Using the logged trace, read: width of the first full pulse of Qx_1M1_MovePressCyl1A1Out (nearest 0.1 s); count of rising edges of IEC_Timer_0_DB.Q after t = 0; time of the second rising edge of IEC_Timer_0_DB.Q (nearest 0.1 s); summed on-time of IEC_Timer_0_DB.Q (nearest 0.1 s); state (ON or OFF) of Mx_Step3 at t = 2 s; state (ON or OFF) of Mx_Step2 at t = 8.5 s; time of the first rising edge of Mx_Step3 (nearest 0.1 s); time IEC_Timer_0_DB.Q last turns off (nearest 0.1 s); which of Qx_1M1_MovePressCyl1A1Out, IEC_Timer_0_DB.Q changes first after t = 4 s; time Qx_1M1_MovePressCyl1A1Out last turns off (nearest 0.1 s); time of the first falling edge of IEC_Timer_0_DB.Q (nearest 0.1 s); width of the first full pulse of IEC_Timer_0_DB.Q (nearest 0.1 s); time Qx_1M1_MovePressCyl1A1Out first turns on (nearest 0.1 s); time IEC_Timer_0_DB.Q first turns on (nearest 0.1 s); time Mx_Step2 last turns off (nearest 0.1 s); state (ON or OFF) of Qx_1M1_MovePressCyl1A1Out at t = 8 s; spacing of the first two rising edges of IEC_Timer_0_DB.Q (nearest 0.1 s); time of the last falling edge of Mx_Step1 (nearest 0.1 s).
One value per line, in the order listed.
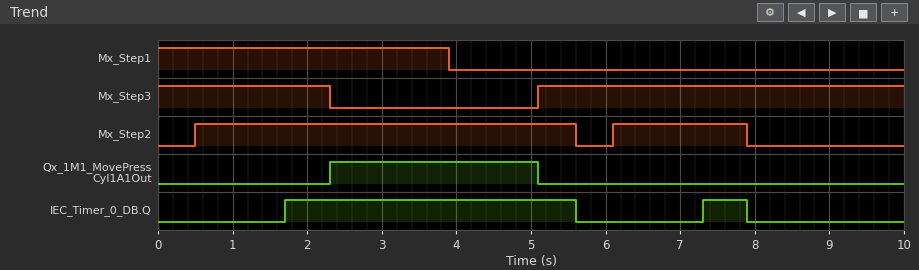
2.8 s
2
7.3 s
4.5 s
ON
OFF
5.1 s
7.9 s
Qx_1M1_MovePressCyl1A1Out
5.1 s
5.6 s
3.9 s
2.3 s
1.7 s
7.9 s
OFF
5.6 s
3.9 s
